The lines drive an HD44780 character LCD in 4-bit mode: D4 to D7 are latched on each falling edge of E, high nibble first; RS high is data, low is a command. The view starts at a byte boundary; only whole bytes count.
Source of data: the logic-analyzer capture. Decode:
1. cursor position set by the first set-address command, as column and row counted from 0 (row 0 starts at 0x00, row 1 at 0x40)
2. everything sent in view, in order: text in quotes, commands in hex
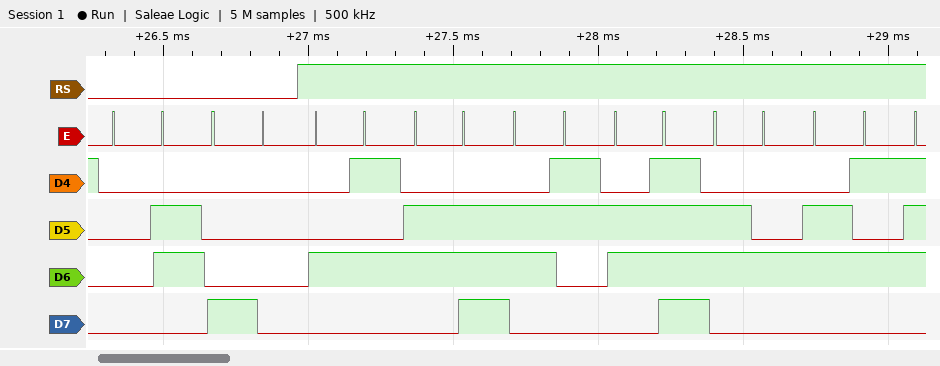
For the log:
column 0, row 0
0x06 0x80 "Encode"
